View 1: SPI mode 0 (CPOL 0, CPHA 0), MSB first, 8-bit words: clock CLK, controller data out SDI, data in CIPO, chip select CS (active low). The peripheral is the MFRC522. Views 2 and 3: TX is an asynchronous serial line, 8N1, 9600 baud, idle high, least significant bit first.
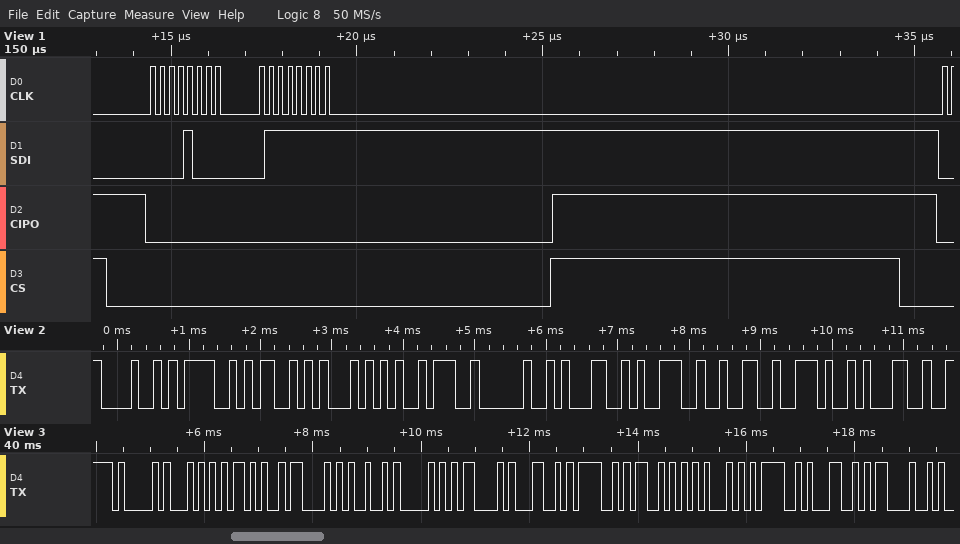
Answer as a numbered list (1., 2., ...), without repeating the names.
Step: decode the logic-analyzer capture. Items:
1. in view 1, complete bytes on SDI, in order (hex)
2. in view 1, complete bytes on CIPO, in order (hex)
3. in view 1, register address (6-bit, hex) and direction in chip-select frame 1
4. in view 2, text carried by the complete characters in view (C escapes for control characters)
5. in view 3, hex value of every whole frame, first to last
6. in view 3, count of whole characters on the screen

1. 0x08 0x7F
2. 0x00 0x00
3. 0x04 write
4. "HOST: 192.1"
5. 0x41 0x54 0x2B 0x43 0x49 0x50 0x43 0x4C 0x4F 0x53 0x45 0x3D 0x31 0x0D
6. 14
